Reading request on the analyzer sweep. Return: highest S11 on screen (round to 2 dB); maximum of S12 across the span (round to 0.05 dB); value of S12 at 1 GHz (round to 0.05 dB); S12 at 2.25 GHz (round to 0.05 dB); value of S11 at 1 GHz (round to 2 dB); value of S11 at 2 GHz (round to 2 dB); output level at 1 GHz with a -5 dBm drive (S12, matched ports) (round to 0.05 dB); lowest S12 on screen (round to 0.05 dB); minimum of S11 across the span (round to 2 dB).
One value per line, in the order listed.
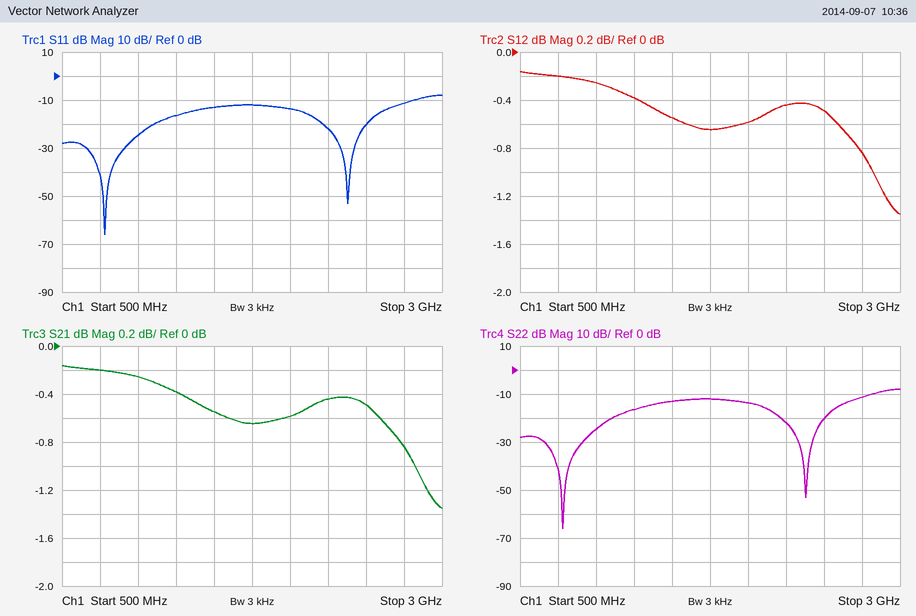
-8 dB
-0.15 dB
-0.25 dB
-0.45 dB
-24 dB
-14 dB
-5.25 dBm
-1.35 dB
-66 dB
